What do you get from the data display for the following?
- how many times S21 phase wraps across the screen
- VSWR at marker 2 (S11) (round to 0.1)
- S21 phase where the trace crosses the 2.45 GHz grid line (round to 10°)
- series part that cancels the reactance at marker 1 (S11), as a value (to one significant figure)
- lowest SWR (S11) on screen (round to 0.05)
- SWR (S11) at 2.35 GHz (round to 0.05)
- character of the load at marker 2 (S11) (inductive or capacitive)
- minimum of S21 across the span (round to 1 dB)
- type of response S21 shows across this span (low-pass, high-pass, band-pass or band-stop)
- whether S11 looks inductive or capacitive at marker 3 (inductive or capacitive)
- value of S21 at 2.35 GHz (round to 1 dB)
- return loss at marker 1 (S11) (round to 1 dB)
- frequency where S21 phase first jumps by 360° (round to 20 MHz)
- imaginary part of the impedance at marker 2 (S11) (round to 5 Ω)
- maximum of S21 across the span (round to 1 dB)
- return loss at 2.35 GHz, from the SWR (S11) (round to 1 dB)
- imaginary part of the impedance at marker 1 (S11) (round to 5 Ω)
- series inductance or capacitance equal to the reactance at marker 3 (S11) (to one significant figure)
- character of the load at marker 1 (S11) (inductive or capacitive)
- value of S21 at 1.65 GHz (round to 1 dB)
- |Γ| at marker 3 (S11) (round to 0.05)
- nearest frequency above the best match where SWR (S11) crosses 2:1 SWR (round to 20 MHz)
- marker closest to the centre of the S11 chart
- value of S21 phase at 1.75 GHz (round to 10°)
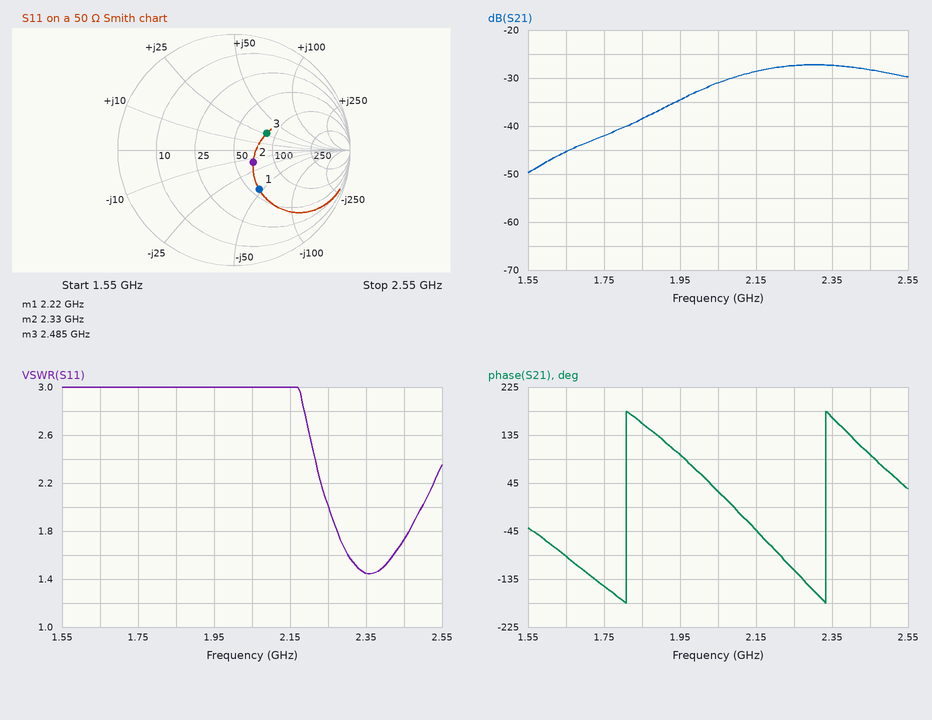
2
1.5
100°
3 nH
1.45
1.45
capacitive
-50 dB
high-pass
inductive
-27 dB
8 dB
1.80 GHz
-15 Ω
-27 dB
15 dB
-45 Ω
2 nH
capacitive
-45 dB
0.30
2.50 GHz
marker 2
-150°
